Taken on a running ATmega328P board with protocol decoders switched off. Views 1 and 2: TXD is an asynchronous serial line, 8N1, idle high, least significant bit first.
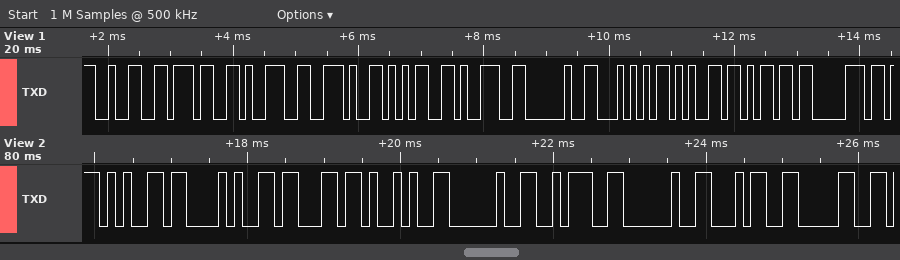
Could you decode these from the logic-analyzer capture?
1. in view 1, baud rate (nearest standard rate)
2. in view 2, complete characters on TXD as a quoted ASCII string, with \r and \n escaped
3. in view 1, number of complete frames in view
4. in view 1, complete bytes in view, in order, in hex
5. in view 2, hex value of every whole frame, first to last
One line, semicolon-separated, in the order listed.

9600 baud; "e(c) : 40"; 11; 0x32 0x37 0x39 0x2E 0x35 0x39 0x20 0x54 0x65 0x6D 0x70; 65 28 63 29 20 3A 20 34 30
